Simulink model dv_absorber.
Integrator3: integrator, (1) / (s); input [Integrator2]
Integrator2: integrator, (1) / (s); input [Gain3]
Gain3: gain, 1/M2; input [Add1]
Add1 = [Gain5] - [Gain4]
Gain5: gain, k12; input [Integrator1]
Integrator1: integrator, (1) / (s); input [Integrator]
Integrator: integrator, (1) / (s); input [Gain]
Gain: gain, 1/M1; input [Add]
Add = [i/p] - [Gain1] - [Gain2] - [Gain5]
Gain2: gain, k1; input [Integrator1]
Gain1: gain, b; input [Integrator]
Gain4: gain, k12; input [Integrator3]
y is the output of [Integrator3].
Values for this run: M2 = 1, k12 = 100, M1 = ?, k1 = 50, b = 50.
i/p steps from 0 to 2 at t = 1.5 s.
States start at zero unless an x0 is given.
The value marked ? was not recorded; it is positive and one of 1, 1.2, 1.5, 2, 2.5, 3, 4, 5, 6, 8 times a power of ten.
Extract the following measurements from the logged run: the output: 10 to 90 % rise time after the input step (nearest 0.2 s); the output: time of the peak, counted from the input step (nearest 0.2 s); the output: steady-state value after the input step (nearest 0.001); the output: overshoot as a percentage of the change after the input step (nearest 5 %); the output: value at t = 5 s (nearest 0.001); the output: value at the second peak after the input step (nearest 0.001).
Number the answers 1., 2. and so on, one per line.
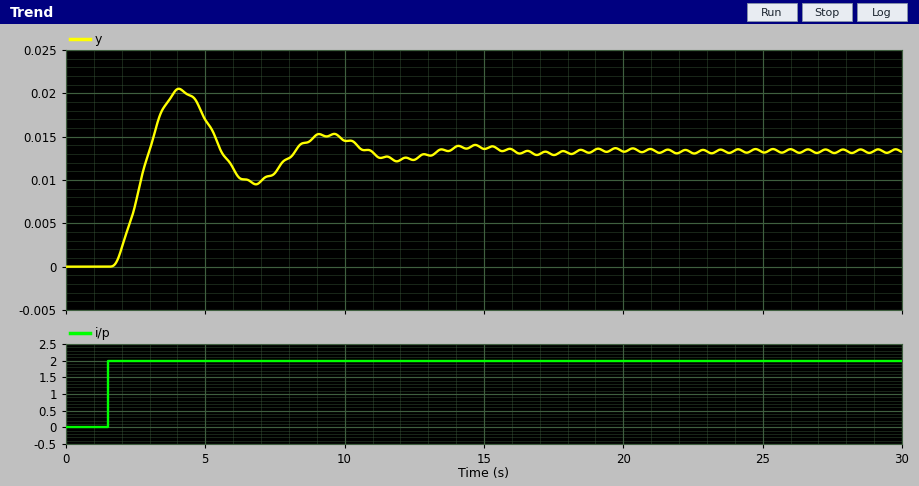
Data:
1. 1.0 s
2. 2.6 s
3. 0.013
4. 55 %
5. 0.017
6. 0.015
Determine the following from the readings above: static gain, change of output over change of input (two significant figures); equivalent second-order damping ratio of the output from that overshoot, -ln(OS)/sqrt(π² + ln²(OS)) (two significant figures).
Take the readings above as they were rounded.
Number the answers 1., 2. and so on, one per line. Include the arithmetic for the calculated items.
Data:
1. (0.013 - 0) / (2 - 0) = 0.0065
2. ln(0.55) = -0.598; 0.598 / sqrt(9.870 + 0.357) = 0.19
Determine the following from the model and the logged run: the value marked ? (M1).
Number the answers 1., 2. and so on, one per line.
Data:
1. 100
